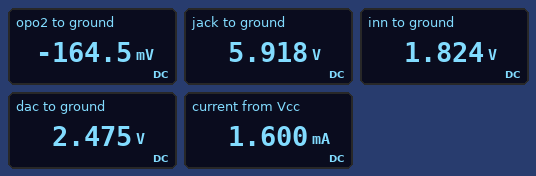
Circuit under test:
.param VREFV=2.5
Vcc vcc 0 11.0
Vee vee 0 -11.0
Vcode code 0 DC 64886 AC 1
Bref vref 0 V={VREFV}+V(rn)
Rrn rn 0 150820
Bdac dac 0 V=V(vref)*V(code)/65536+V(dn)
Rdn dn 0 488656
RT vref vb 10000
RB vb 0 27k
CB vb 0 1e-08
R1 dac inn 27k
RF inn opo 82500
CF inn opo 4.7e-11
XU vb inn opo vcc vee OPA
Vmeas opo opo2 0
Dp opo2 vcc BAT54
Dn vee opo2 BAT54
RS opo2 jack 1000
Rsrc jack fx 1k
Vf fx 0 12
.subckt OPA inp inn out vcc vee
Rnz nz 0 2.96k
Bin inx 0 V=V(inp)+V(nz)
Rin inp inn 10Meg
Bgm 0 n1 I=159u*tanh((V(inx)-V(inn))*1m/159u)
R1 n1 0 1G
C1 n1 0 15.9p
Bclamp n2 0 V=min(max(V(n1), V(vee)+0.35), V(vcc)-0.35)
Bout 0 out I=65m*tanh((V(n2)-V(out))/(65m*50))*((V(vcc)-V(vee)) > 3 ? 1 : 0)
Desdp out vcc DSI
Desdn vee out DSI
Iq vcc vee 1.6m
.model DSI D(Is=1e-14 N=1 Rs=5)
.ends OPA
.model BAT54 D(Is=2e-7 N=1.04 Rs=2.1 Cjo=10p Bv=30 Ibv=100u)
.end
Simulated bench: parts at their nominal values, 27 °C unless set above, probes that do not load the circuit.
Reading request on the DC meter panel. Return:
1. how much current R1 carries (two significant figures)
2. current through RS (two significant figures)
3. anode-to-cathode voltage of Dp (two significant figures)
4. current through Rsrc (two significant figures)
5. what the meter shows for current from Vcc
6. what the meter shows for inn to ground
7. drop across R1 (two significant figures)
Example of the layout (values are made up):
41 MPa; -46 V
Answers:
24 µA; 6.1 mA; -11 V; 6.1 mA; 1.600 mA; 1.824 V; 650 mV
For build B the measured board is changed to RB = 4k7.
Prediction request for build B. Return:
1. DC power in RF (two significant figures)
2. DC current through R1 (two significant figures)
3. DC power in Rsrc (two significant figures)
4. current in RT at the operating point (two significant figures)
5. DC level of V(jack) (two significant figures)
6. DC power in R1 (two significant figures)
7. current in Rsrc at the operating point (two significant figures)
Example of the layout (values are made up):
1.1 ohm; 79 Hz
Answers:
320 µW; 62 µA; 67 mW; 170 µA; 3.8 V; 100 µW; 8.2 mA
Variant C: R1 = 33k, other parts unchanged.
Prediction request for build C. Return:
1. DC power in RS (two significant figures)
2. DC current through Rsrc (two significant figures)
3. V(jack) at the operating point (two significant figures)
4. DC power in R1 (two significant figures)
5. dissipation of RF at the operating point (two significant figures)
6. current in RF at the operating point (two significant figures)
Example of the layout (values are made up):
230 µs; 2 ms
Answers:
35 mW; 5.9 mA; 6.1 V; 13 µW; 32 µW; 20 µA
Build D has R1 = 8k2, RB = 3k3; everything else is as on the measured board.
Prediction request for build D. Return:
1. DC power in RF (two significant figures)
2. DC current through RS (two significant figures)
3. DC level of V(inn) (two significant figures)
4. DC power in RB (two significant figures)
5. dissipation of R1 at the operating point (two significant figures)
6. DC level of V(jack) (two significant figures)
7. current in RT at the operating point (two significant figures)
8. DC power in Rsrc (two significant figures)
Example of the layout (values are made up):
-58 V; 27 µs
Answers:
1.6 mW; 11 mA; 1.3 V; 120 µW; 160 µW; 960 mV; 190 µA; 120 mW
